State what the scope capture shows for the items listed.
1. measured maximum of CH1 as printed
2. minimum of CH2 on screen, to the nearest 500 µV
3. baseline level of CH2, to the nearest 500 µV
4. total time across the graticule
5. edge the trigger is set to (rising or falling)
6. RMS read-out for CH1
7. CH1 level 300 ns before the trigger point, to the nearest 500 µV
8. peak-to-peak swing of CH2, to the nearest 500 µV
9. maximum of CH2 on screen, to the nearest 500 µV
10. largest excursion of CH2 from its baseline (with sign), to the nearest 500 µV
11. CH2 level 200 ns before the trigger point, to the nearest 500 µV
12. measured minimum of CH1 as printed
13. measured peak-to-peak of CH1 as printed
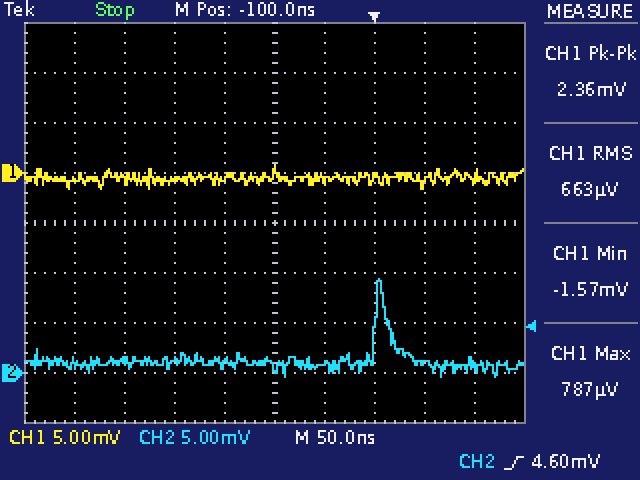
787 µV
-500 µV
1.0 mV
500 ns
rising
663 µV
-500 µV
10.0 mV
9.5 mV
+8.5 mV
1.0 mV
-1.57 mV
2.36 mV
